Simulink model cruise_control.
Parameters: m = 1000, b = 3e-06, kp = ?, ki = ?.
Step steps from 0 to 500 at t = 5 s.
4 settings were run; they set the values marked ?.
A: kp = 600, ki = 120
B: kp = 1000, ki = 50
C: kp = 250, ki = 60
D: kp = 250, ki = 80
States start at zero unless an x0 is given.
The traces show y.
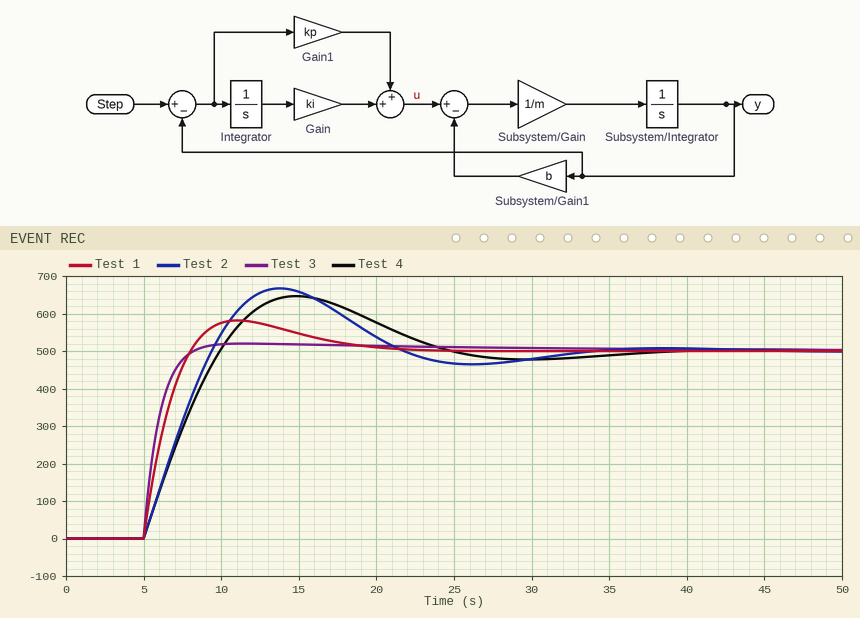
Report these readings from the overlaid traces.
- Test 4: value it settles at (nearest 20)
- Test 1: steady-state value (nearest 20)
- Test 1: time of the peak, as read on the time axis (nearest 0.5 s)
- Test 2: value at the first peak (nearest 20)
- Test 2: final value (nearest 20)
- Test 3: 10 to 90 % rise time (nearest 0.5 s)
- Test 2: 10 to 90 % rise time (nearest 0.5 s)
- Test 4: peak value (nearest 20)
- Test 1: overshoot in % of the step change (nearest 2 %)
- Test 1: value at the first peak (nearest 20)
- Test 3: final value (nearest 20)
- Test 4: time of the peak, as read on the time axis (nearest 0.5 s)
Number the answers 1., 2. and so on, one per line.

1. 500
2. 500
3. 11.0 s
4. 660
5. 500
6. 2.0 s
7. 3.5 s
8. 640
9. 16 %
10. 580
11. 500
12. 15.0 s
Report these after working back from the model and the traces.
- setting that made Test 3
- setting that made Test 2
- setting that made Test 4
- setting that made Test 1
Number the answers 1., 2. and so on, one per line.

1. B
2. D
3. C
4. A
